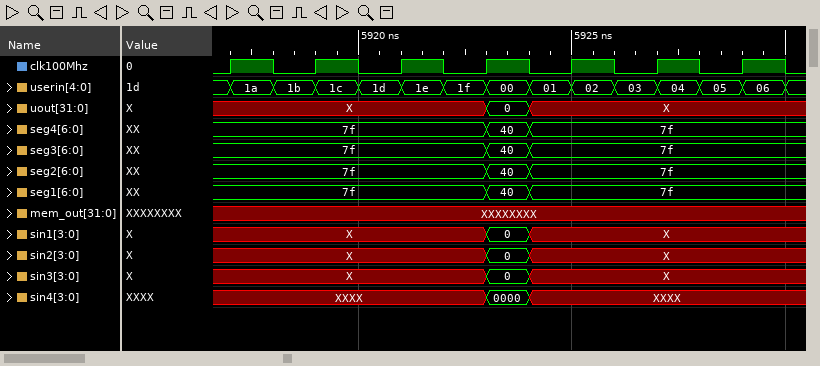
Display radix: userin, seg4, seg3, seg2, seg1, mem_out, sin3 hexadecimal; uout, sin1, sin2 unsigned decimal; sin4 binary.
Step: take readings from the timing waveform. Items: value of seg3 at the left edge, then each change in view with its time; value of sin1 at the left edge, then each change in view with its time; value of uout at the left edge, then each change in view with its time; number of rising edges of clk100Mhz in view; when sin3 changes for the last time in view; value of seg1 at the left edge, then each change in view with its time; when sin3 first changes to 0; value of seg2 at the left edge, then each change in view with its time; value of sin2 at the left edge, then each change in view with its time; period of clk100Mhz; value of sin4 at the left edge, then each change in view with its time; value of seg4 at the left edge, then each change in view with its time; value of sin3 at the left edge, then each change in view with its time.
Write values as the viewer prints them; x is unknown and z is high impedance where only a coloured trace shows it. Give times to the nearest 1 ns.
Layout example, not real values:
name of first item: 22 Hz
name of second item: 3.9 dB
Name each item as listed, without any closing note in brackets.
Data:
value of seg3 at the left edge, then each change in view with its time: 7f, 40 at 5923 ns, 7f at 5924 ns
value of sin1 at the left edge, then each change in view with its time: X, 0 at 5923 ns, X at 5924 ns
value of uout at the left edge, then each change in view with its time: X, 0 at 5923 ns, X at 5924 ns
number of rising edges of clk100Mhz in view: 7
when sin3 changes for the last time in view: 5924 ns
value of seg1 at the left edge, then each change in view with its time: 7f, 40 at 5923 ns, 7f at 5924 ns
when sin3 first changes to 0: 5923 ns
value of seg2 at the left edge, then each change in view with its time: 7f, 40 at 5923 ns, 7f at 5924 ns
value of sin2 at the left edge, then each change in view with its time: X, 0 at 5923 ns, X at 5924 ns
period of clk100Mhz: 2 ns
value of sin4 at the left edge, then each change in view with its time: XXXX, 0000 at 5923 ns, XXXX at 5924 ns
value of seg4 at the left edge, then each change in view with its time: 7f, 40 at 5923 ns, 7f at 5924 ns
value of sin3 at the left edge, then each change in view with its time: X, 0 at 5923 ns, X at 5924 ns
